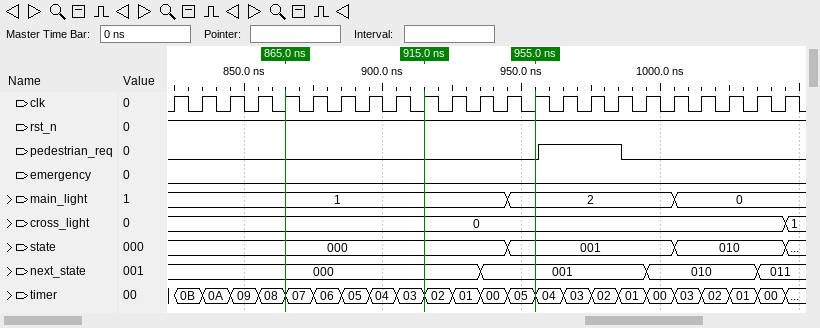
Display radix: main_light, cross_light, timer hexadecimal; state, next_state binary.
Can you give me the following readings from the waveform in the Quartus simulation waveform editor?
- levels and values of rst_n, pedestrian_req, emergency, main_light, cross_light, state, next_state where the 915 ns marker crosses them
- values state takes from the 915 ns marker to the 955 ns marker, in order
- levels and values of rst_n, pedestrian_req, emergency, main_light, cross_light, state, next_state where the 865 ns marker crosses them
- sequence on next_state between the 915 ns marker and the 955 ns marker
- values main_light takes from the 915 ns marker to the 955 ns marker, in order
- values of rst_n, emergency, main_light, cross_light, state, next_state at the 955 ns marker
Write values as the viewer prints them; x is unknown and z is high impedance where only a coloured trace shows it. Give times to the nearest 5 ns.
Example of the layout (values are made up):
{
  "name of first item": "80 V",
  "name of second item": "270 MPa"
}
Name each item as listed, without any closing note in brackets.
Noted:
{
  "levels and values of rst_n, pedestrian_req, emergency, main_light, cross_light, state, next_state where the 915 ns marker crosses them": "rst_n=1, pedestrian_req=0, emergency=0, main_light=1, cross_light=0, state=000, next_state=000",
  "values state takes from the 915 ns marker to the 955 ns marker, in order": "000, 001",
  "levels and values of rst_n, pedestrian_req, emergency, main_light, cross_light, state, next_state where the 865 ns marker crosses them": "rst_n=1, pedestrian_req=0, emergency=0, main_light=1, cross_light=0, state=000, next_state=000",
  "sequence on next_state between the 915 ns marker and the 955 ns marker": "000, 001",
  "values main_light takes from the 915 ns marker to the 955 ns marker, in order": "1, 2",
  "values of rst_n, emergency, main_light, cross_light, state, next_state at the 955 ns marker": "rst_n=1, emergency=0, main_light=2, cross_light=0, state=001, next_state=001"
}
